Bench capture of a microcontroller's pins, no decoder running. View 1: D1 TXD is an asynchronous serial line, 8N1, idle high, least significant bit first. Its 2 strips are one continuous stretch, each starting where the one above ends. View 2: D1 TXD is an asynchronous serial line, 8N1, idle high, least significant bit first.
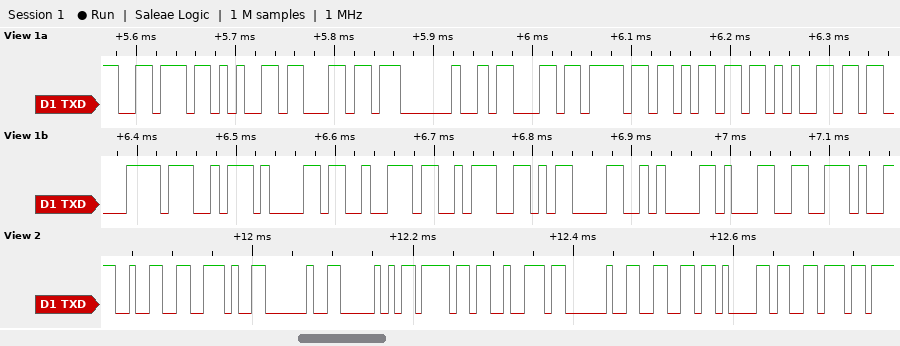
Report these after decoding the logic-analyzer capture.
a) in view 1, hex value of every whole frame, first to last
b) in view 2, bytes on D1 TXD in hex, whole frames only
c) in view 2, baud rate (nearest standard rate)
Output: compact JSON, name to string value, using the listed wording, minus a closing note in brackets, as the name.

{"in view 1, hex value of every whole frame, first to last": "76 65 6C 20 63 6F 6D 65 C3 A7 61 72 3A 0D 0A 31 2E", "in view 2, bytes on D1 TXD in hex, whole frames only": "32 2E 20 50 6F 72 20 66 61 76", "in view 2, baud rate": "115200 baud"}
